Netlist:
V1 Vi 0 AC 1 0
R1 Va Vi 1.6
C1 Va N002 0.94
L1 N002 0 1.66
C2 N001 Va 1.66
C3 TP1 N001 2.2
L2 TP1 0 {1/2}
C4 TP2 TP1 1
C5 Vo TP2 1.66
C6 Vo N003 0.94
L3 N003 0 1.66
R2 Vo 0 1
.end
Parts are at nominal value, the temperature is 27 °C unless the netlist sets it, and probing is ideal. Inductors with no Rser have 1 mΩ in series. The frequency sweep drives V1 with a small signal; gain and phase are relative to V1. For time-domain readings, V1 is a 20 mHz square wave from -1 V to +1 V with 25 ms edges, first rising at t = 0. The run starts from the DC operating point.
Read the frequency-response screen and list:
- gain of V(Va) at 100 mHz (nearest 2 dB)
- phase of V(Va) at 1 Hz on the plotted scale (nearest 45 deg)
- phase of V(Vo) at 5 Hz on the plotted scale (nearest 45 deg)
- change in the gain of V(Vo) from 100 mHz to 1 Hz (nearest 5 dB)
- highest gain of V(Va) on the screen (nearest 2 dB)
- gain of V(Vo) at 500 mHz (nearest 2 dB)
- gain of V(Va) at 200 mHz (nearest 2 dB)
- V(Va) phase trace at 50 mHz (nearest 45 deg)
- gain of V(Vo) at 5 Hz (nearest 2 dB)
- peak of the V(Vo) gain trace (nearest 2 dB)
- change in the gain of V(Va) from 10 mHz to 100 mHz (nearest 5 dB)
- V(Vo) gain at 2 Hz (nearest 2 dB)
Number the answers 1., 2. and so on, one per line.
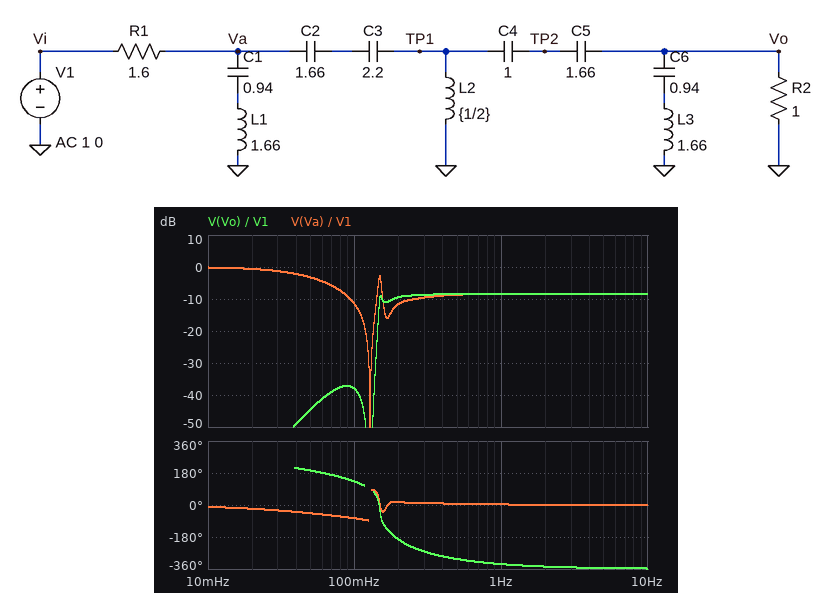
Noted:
1. -12 dB
2. 0 deg
3. -360 deg
4. 30 dB
5. 0 dB
6. -8 dB
7. -12 dB
8. -45 deg
9. -8 dB
10. -8 dB
11. -10 dB
12. -8 dB
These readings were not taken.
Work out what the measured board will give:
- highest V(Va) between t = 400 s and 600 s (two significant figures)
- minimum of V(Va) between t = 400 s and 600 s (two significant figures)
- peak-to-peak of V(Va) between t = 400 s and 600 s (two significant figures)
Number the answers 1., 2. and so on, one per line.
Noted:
1. 1.0 V
2. -1.0 V
3. 2.1 V
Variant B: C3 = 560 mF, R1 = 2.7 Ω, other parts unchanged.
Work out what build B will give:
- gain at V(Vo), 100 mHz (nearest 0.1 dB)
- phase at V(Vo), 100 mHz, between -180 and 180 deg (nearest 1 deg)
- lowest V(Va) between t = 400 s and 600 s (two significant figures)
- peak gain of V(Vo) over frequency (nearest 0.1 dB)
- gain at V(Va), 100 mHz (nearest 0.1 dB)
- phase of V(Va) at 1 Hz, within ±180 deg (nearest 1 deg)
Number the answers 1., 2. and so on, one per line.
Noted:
1. -48.8 dB
2. 128 deg
3. -1.0 V
4. -10.4 dB
5. -14.0 dB
6. -5 deg
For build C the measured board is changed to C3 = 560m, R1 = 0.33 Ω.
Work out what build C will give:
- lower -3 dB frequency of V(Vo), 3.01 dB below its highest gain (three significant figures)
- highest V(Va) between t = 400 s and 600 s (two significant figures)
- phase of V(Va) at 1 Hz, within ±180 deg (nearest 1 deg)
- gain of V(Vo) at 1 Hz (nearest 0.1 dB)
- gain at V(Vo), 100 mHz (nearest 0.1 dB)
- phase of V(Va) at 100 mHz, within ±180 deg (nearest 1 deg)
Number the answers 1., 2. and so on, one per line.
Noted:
1. 195 mHz
2. 1.3 V
3. -2 deg
4. -2.6 dB
5. -36.1 dB
6. -31 deg
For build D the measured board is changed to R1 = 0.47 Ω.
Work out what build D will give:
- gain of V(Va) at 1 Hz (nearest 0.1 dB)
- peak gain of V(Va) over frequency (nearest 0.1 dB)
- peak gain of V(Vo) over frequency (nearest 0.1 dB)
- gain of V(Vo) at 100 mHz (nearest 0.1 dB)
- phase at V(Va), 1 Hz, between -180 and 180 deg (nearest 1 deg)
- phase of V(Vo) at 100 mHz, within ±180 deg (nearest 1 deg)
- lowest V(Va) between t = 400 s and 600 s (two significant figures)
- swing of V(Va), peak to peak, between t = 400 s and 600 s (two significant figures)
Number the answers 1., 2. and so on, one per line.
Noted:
1. -3.4 dB
2. 0 dB
3. -2.9 dB
4. -29.8 dB
5. 2 deg
6. 159 deg
7. -1.2 V
8. 2.4 V
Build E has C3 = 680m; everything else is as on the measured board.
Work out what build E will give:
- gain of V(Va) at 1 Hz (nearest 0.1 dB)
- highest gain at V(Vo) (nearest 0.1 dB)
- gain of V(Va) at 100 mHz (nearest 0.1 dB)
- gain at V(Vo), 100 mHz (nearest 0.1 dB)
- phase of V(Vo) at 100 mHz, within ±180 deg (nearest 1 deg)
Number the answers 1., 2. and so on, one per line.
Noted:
1. -8.2 dB
2. -8.1 dB
3. -10.0 dB
4. -43.4 dB
5. 135 deg
